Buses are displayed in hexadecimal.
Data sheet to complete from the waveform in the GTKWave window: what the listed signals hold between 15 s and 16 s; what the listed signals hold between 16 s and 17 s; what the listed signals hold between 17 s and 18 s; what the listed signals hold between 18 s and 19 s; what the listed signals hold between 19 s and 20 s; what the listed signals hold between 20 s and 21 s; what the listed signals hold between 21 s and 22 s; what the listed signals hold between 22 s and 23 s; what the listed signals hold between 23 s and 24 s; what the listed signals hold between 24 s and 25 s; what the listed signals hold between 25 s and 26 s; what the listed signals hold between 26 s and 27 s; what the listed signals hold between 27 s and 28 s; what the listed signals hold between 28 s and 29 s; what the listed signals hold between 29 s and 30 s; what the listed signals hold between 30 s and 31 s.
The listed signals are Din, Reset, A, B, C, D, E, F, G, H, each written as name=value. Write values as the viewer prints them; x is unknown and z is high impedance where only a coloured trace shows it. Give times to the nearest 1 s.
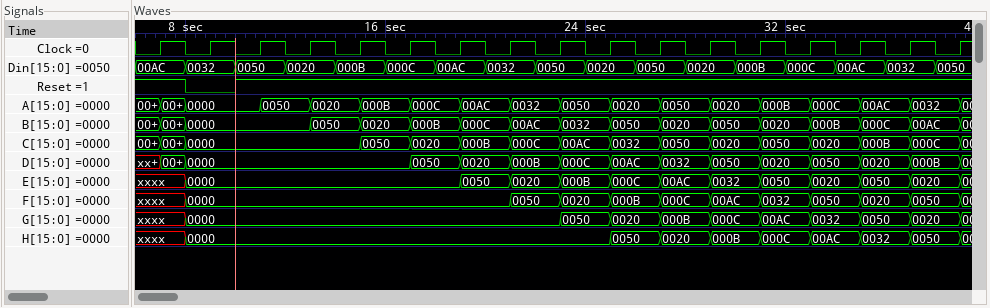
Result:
Din=000B, Reset=1, A=000B, B=0020, C=0050, D=0000, E=0000, F=0000, G=0000, H=0000
Din=000C, Reset=1, A=000B, B=0020, C=0050, D=0000, E=0000, F=0000, G=0000, H=0000
Din=000C, Reset=1, A=000C, B=000B, C=0020, D=0050, E=0000, F=0000, G=0000, H=0000
Din=00AC, Reset=1, A=000C, B=000B, C=0020, D=0050, E=0000, F=0000, G=0000, H=0000
Din=00AC, Reset=1, A=00AC, B=000C, C=000B, D=0020, E=0050, F=0000, G=0000, H=0000
Din=0032, Reset=1, A=00AC, B=000C, C=000B, D=0020, E=0050, F=0000, G=0000, H=0000
Din=0032, Reset=1, A=0032, B=00AC, C=000C, D=000B, E=0020, F=0050, G=0000, H=0000
Din=0050, Reset=1, A=0032, B=00AC, C=000C, D=000B, E=0020, F=0050, G=0000, H=0000
Din=0050, Reset=1, A=0050, B=0032, C=00AC, D=000C, E=000B, F=0020, G=0050, H=0000
Din=0020, Reset=1, A=0050, B=0032, C=00AC, D=000C, E=000B, F=0020, G=0050, H=0000
Din=0020, Reset=1, A=0020, B=0050, C=0032, D=00AC, E=000C, F=000B, G=0020, H=0050
Din=0050, Reset=1, A=0020, B=0050, C=0032, D=00AC, E=000C, F=000B, G=0020, H=0050
Din=0050, Reset=1, A=0050, B=0020, C=0050, D=0032, E=00AC, F=000C, G=000B, H=0020
Din=0020, Reset=1, A=0050, B=0020, C=0050, D=0032, E=00AC, F=000C, G=000B, H=0020
Din=0020, Reset=1, A=0020, B=0050, C=0020, D=0050, E=0032, F=00AC, G=000C, H=000B
Din=000B, Reset=1, A=0020, B=0050, C=0020, D=0050, E=0032, F=00AC, G=000C, H=000B
